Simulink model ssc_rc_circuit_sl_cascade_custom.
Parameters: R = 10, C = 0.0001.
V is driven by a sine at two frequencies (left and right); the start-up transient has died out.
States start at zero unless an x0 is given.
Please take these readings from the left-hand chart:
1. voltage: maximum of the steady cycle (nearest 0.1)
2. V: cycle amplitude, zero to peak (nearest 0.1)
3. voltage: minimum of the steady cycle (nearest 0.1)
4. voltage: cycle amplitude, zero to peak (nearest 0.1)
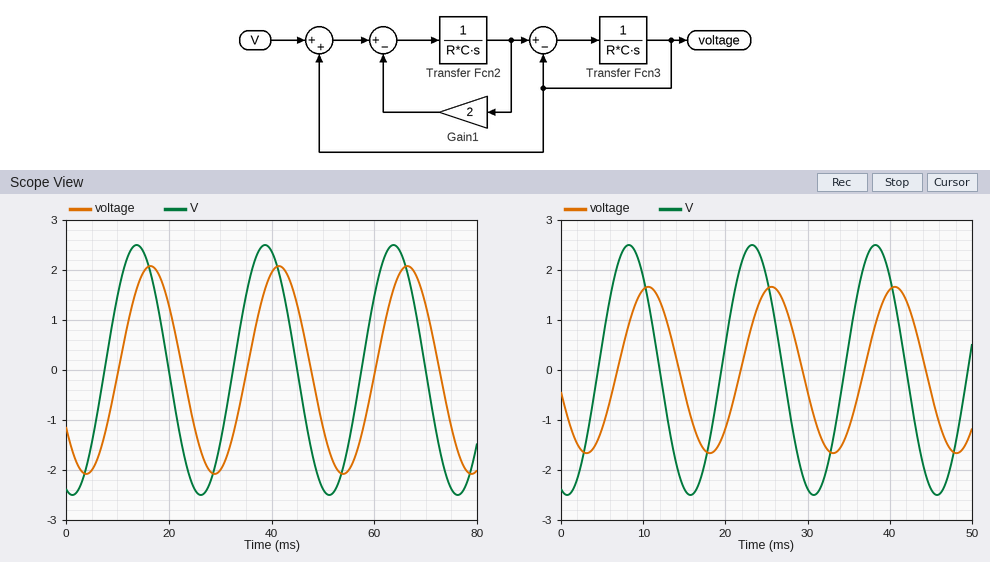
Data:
2.1
2.5
-2.1
2.1
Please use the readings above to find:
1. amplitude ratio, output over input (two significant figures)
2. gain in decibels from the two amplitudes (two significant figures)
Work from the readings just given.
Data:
0.84
-1.5 dB
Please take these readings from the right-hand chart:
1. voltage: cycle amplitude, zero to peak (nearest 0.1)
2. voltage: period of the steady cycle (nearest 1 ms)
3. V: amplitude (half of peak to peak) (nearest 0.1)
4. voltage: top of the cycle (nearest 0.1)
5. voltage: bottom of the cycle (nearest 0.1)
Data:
1.7
15 ms
2.5
1.7
-1.7
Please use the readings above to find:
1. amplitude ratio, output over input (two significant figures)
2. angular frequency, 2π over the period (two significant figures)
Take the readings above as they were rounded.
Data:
0.68
0.42 rad/ms
